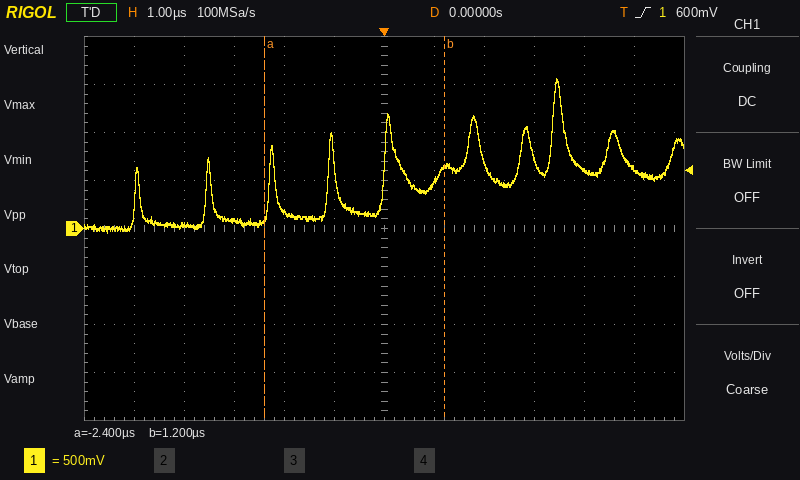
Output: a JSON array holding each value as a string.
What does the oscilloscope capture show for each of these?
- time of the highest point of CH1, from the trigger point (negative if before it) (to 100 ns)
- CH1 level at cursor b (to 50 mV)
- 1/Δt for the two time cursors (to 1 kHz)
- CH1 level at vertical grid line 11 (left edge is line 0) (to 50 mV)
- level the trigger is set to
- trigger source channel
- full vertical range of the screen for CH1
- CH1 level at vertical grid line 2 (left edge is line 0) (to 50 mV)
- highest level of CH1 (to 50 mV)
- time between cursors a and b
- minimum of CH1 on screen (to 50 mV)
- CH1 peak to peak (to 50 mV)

["+3.5 µs", "650 mV", "278 kHz", "600 mV", "600 mV", "CH1", "4 V", "50 mV", "1.55 V", "3.6 µs", "-50 mV", "1.60 V"]
